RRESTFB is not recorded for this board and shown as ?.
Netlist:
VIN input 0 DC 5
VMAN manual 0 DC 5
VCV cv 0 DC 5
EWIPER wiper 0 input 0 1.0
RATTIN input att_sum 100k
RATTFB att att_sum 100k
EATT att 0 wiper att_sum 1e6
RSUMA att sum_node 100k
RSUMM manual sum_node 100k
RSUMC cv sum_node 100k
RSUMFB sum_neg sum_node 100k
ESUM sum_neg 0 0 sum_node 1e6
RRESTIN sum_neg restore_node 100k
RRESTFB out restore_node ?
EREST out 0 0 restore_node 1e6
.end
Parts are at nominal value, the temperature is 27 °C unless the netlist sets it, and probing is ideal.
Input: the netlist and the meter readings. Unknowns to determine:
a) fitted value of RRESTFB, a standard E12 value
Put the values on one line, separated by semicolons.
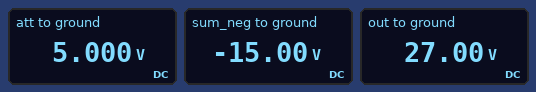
180 kΩ
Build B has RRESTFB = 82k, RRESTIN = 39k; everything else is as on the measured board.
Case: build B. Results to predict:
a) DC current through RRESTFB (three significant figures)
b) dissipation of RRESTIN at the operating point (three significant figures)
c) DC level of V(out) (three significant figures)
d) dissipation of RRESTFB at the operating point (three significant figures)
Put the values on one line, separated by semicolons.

385 µA; 5.77 mW; 31.5 V; 12.1 mW
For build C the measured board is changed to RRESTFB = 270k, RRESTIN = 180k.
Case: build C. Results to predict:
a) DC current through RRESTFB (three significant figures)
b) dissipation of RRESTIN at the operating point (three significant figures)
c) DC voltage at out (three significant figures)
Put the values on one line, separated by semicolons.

83.3 µA; 1.25 mW; 22.5 V
